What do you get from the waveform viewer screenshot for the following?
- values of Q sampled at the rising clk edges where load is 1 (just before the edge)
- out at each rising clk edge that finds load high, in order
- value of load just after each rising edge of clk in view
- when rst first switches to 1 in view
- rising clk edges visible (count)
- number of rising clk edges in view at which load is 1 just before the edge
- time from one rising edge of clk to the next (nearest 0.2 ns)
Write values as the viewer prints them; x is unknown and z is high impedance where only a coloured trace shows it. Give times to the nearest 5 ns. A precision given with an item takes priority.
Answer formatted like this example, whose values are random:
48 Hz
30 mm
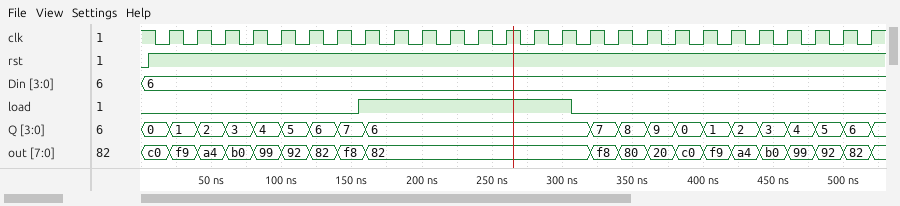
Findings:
7, 6, 6, 6, 6, 6, 6, 6
f8, 82, 82, 82, 82, 82, 82, 82
0 0 0 0 0 0 0 1 1 1 1 1 1 1 1 0 0 0 0 0 0 0 0 0 0 0
5 ns
26
8
20 ns
